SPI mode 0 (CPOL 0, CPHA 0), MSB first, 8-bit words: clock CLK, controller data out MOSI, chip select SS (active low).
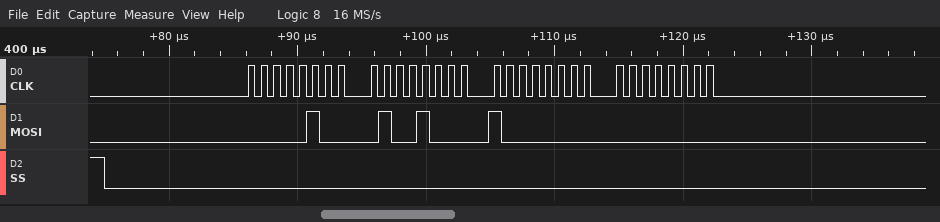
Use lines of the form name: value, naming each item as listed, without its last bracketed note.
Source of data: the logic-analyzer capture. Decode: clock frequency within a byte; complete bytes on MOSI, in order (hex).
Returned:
clock frequency within a byte: 1 MHz
complete bytes on MOSI, in order: 04 48 80 00
